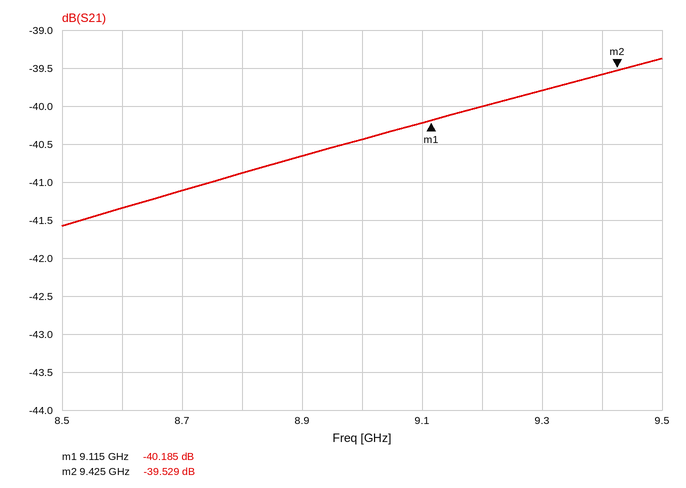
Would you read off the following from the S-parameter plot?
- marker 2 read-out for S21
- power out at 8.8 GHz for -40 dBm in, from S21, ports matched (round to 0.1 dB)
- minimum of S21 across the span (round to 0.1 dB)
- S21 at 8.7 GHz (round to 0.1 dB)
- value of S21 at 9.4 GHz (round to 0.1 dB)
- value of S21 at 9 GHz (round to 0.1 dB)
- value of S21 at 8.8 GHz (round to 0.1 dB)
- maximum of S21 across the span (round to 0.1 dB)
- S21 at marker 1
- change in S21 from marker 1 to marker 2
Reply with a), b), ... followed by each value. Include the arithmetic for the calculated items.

a) -39.529 dB
b) -40 dBm + (-40.9 dB) = -80.9 dBm
c) -41.6 dB
d) -41.1 dB
e) -39.6 dB
f) -40.4 dB
g) -40.9 dB
h) -39.4 dB
i) -40.185 dB
j) -39.529 − (-40.185) = 0.656 dB
